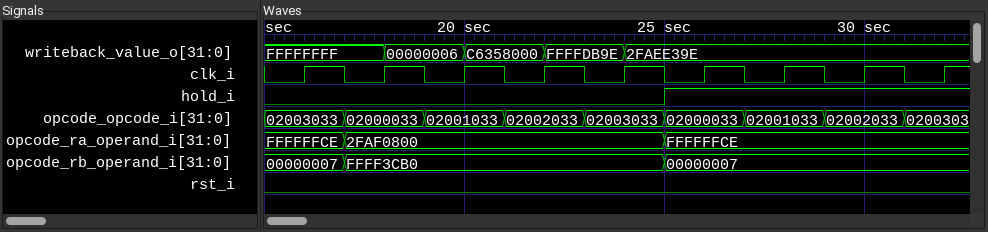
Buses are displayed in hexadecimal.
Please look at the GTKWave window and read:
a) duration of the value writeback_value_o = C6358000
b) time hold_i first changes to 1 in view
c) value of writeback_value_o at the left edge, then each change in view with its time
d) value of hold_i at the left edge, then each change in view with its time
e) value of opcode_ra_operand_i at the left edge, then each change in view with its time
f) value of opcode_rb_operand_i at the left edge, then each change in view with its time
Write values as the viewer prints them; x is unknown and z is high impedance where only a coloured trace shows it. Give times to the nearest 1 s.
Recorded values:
2 s
25 s
FFFFFFFF, 00000006 at 18 s, C6358000 at 20 s, FFFFDB9E at 22 s, 2FAEE39E at 24 s
0, 1 at 25 s
FFFFFFCE, 2FAF0800 at 17 s, FFFFFFCE at 25 s
00000007, FFFF3CB0 at 17 s, 00000007 at 25 s
